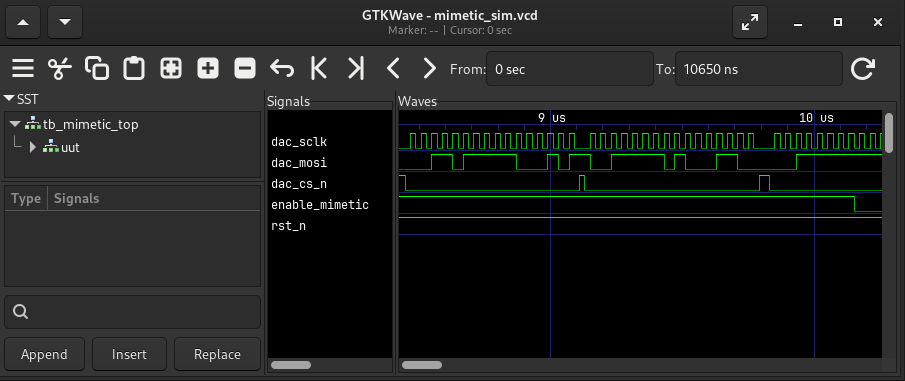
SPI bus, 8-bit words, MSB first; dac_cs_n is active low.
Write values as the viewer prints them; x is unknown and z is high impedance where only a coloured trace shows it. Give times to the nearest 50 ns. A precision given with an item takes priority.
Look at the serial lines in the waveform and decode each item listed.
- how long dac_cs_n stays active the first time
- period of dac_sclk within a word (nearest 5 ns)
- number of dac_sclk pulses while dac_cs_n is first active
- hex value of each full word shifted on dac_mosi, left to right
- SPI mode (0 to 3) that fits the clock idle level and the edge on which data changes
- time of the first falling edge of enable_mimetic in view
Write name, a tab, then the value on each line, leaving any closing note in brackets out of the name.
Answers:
how long dac_cs_n stays active the first time	650 ns
period of dac_sclk within a word	40 ns
number of dac_sclk pulses while dac_cs_n is first active	16
hex value of each full word shifted on dac_mosi, left to right	37, C5, 3E, 8C, 3F
SPI mode (0 to 3) that fits the clock idle level and the edge on which data changes	1
time of the first falling edge of enable_mimetic in view	10150 ns
